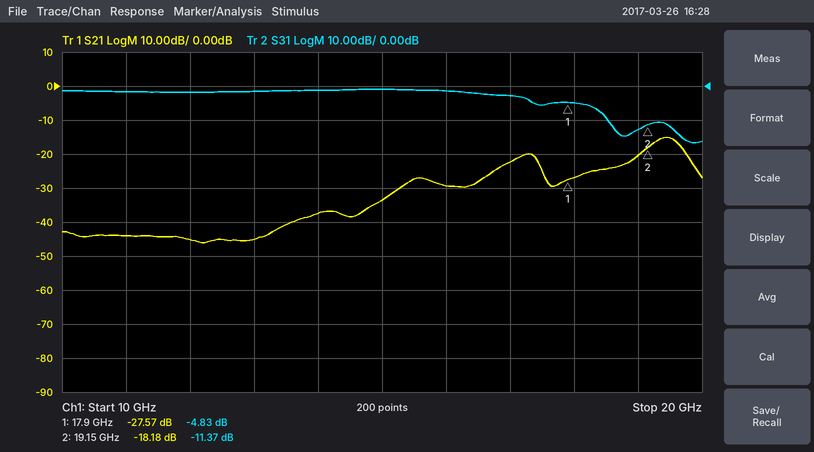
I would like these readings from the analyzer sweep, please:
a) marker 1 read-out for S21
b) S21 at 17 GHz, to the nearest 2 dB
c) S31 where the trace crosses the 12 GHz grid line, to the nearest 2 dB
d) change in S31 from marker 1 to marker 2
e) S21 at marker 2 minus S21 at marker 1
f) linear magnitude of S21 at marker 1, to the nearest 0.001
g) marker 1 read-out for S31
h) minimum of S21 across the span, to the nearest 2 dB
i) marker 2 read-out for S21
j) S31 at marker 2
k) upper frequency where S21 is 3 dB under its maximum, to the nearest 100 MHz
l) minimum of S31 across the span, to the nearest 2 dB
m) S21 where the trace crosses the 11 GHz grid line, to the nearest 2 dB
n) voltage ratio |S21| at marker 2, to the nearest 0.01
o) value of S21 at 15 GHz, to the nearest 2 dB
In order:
-27.57 dB
-22 dB
-2 dB
-6.54 dB
9.39 dB
0.042
-4.83 dB
-46 dB
-18.18 dB
-11.37 dB
19.7 GHz
-16 dB
-44 dB
0.12
-34 dB
